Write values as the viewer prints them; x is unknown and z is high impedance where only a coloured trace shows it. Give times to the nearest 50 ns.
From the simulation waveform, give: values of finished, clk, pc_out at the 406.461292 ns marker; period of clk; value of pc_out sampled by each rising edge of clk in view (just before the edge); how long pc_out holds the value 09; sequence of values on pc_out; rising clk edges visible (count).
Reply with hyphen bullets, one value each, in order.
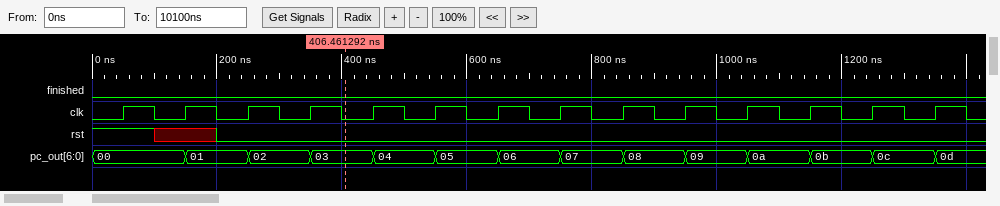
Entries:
- finished=0, clk=0, pc_out=03
- 100 ns
- 00, 00, 01, 02, 03, 04, 05, 06, 07, 08, 09, 0a, 0b, 0c
- 100 ns
- 00, 01, 02, 03, 04, 05, 06, 07, 08, 09, 0a, 0b, 0c, 0d
- 14
